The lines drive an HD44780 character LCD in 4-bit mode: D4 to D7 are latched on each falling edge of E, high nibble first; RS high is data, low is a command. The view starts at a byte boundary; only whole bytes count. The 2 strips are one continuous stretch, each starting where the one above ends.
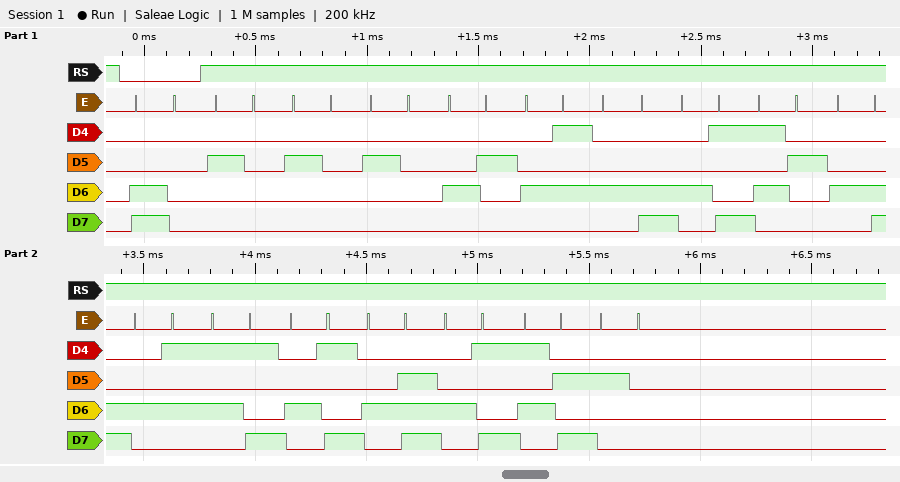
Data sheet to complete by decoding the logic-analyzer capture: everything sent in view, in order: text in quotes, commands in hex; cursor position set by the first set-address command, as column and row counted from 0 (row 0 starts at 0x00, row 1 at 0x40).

0xC0 "   BELIRLEYINIZ "
column 0, row 1
